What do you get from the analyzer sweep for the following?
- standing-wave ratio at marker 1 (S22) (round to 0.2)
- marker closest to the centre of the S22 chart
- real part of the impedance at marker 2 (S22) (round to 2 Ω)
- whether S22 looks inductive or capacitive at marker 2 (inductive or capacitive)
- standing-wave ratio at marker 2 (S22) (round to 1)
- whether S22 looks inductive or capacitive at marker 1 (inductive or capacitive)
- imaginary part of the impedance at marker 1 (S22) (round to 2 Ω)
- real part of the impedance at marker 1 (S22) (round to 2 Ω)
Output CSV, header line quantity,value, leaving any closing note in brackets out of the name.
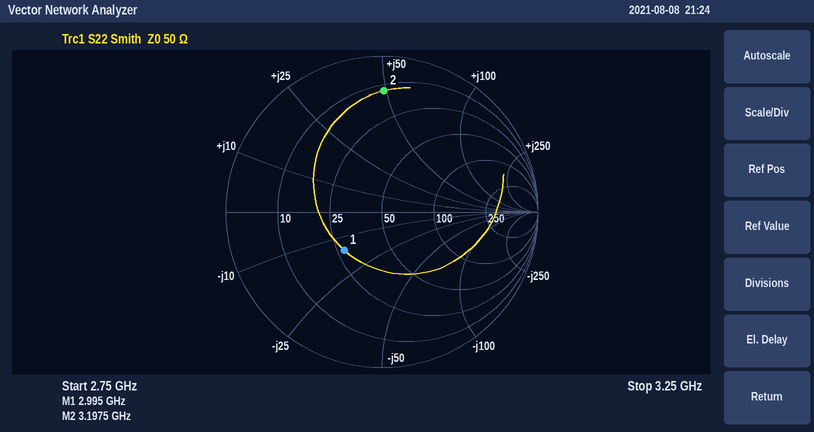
quantity,value
standing-wave ratio at marker 1 (S22),2.0
marker closest to the centre of the S22 chart,marker 1
real part of the impedance at marker 2 (S22),12 Ω
whether S22 looks inductive or capacitive at marker 2,inductive
standing-wave ratio at marker 2 (S22),8
whether S22 looks inductive or capacitive at marker 1,capacitive
imaginary part of the impedance at marker 1 (S22),-16 Ω
real part of the impedance at marker 1 (S22),28 Ω
